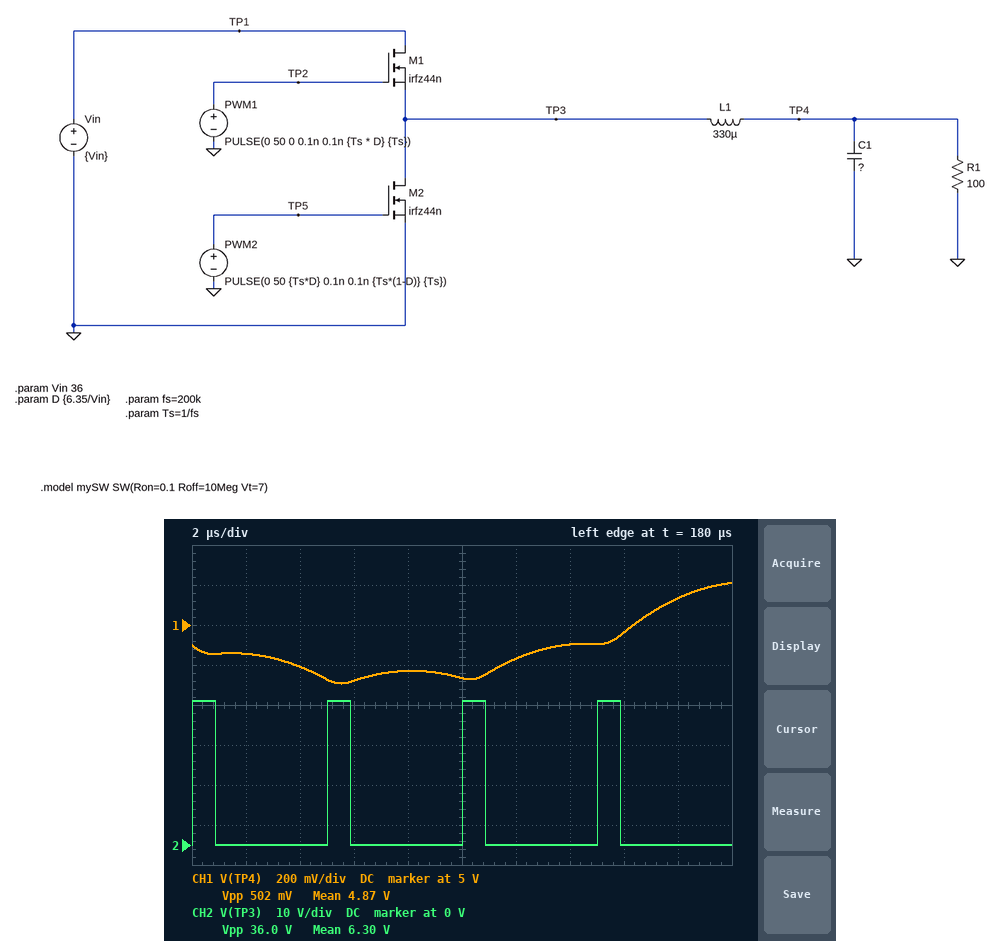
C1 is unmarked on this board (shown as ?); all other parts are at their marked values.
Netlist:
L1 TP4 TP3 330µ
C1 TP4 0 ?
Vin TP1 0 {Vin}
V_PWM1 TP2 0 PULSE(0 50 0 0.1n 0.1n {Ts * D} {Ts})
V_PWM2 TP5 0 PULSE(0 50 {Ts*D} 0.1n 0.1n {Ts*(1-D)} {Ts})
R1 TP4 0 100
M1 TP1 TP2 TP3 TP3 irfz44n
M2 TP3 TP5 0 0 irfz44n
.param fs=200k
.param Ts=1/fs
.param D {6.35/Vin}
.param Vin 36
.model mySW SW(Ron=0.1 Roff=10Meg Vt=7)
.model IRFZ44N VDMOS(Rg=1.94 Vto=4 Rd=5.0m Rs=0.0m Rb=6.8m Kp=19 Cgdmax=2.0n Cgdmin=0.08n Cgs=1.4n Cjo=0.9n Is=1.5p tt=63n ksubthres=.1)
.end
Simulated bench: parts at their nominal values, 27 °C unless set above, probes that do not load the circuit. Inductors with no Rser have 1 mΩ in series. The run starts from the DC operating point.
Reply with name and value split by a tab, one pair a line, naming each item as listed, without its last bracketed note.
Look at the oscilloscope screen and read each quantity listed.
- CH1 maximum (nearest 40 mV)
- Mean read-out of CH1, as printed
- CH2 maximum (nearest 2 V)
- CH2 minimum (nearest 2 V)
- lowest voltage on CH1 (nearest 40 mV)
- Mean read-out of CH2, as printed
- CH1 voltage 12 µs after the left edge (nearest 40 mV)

CH1 maximum	5.20 V
Mean read-out of CH1, as printed	4.87 V
CH2 maximum	36 V
CH2 minimum	0 V
lowest voltage on CH1	4.72 V
Mean read-out of CH2, as printed	6.30 V
CH1 voltage 12 µs after the left edge	4.84 V
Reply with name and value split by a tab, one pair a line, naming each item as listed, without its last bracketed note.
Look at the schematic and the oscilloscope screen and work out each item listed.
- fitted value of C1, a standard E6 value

fitted value of C1, a standard E6 value	680 nF
